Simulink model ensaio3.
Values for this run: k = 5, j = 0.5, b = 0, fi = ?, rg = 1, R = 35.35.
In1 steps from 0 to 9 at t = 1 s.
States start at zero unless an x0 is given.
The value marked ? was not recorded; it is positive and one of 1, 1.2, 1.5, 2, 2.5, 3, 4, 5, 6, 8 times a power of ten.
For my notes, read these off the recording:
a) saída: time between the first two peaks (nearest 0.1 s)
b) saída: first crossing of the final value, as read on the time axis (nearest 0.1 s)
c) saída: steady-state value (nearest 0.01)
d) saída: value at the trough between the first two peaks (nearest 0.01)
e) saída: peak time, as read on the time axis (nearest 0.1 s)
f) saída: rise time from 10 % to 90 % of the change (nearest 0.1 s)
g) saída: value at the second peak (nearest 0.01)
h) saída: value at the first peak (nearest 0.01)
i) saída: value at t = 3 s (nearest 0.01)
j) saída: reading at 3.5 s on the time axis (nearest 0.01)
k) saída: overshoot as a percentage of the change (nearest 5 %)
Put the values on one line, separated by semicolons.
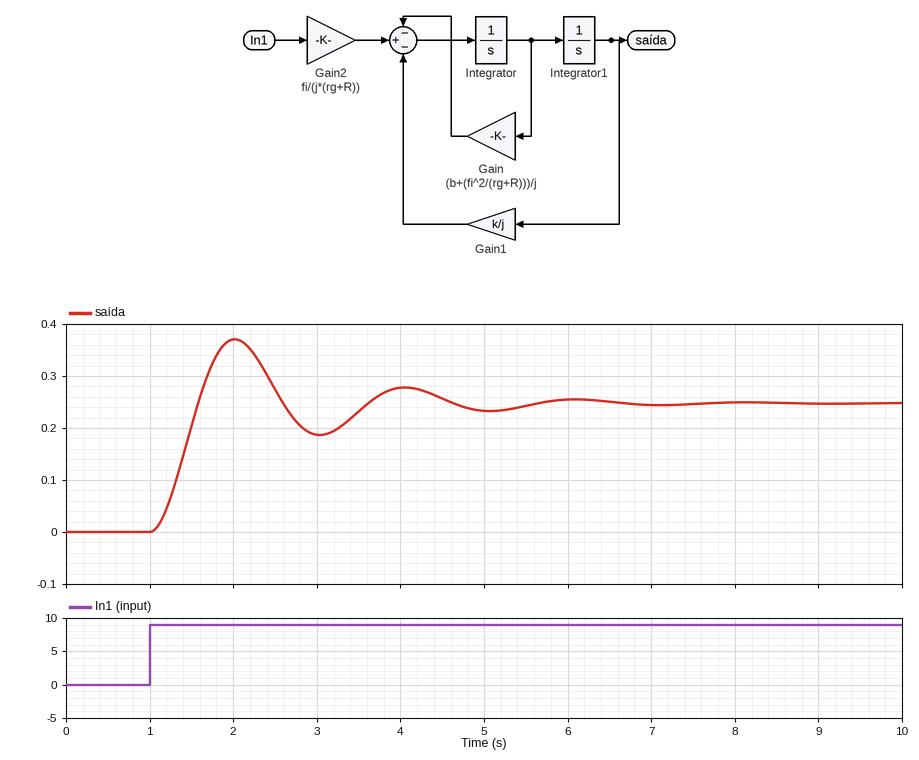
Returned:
2.0 s; 1.6 s; 0.25; 0.19; 2.0 s; 0.4 s; 0.28; 0.37; 0.19; 0.23; 50 %
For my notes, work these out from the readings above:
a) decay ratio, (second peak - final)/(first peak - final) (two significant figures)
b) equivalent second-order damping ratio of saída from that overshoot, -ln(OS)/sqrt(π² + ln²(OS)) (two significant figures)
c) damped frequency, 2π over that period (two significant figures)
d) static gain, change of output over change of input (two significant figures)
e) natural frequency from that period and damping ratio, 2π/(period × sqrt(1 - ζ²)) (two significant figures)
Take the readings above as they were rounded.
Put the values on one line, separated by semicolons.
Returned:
0.25; 0.22; 3.1 rad/s; 0.028; 3.2 rad/s
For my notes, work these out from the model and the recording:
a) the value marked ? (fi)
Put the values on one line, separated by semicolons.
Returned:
5
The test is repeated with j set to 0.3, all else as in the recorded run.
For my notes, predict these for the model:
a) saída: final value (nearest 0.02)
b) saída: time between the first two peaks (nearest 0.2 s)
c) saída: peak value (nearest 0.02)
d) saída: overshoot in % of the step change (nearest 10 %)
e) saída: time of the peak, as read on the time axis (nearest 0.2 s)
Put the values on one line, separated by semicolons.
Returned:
0.24; 1.6 s; 0.34; 40 %; 1.8 s
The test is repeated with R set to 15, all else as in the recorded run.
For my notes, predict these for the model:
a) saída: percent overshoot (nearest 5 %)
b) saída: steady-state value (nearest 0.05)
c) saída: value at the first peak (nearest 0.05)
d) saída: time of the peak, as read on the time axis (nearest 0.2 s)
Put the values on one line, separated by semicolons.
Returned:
15 %; 0.55; 0.65; 2.2 s
